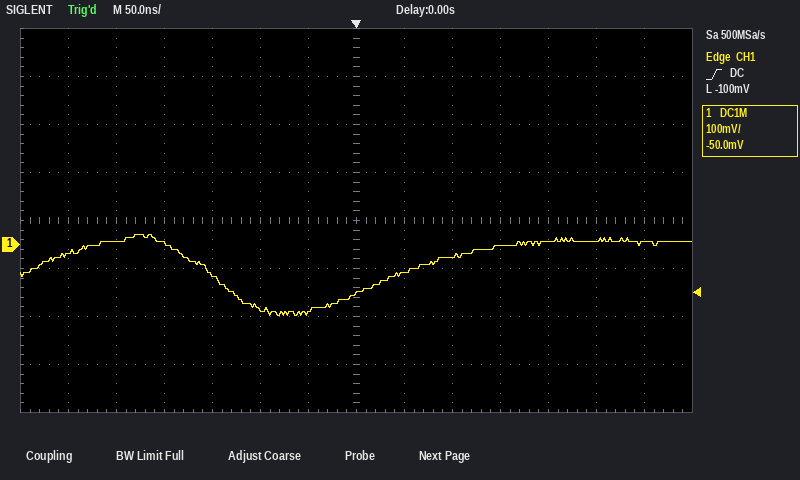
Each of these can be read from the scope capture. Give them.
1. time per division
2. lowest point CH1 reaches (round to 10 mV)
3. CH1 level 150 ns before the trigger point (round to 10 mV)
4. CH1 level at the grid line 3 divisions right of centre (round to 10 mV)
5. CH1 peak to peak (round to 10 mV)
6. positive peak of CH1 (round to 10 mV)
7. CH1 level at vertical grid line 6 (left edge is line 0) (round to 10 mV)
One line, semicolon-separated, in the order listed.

50 ns; -150 mV; -60 mV; 0 mV; 170 mV; 20 mV; -140 mV
